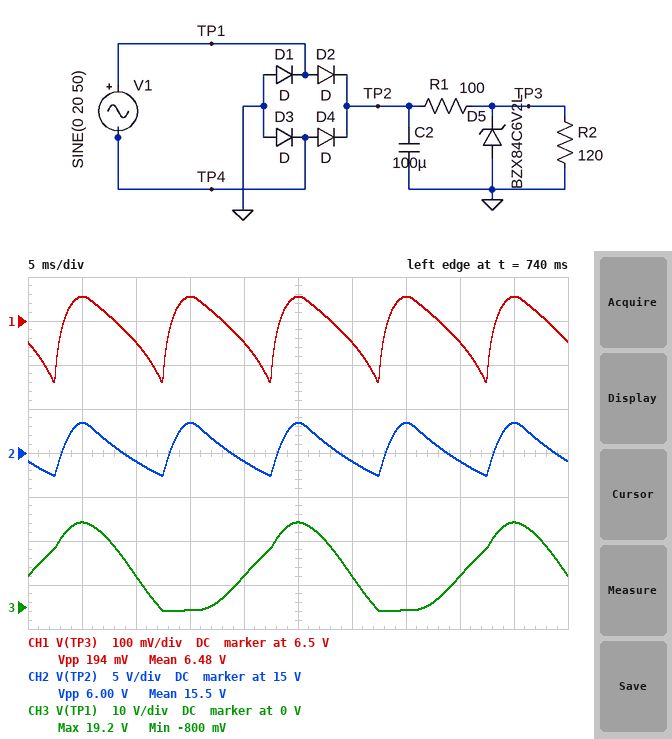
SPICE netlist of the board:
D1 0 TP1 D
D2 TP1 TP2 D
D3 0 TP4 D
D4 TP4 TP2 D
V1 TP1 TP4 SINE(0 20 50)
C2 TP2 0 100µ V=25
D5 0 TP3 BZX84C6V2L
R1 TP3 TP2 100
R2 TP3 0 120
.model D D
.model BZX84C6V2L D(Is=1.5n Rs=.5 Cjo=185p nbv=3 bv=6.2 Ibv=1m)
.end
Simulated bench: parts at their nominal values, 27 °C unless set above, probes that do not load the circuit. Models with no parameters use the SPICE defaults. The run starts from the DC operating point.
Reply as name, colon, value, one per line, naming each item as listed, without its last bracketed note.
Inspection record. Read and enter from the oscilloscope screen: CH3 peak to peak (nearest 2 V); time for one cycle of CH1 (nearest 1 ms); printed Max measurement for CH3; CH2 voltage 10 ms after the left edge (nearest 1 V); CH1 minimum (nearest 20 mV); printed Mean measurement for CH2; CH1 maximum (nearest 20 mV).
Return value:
CH3 peak to peak: 20 V
time for one cycle of CH1: 10 ms
printed Max measurement for CH3: 19.2 V
CH2 voltage 10 ms after the left edge: 14 V
CH1 minimum: 6.36 V
printed Mean measurement for CH2: 15.5 V
CH1 maximum: 6.56 V
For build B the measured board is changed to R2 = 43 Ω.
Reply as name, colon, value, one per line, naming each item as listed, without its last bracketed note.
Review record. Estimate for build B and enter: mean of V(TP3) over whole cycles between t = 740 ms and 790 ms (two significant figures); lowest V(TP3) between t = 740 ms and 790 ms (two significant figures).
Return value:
mean of V(TP3) over whole cycles between t = 740 ms and 790 ms: 4.6 V
lowest V(TP3) between t = 740 ms and 790 ms: 3.4 V
